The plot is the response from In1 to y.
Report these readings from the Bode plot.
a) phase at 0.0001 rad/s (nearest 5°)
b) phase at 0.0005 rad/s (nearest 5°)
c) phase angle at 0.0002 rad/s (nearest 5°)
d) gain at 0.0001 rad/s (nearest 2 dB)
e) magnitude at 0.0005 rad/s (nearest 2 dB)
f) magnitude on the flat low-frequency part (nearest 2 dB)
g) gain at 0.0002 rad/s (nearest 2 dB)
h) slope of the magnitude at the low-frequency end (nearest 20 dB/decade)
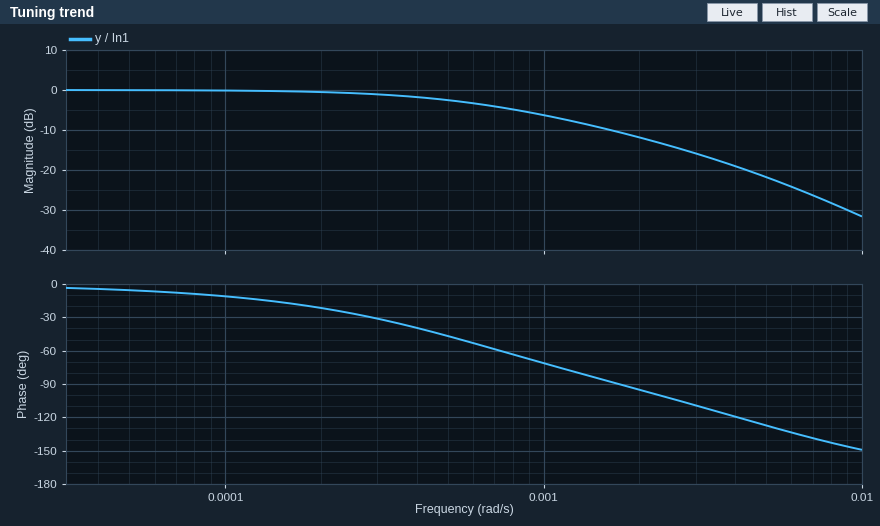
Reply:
-10°
-45°
-20°
0 dB
-2 dB
0 dB
0 dB
0 dB/decade
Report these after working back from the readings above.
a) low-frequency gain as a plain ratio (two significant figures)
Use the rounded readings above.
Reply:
1.0
